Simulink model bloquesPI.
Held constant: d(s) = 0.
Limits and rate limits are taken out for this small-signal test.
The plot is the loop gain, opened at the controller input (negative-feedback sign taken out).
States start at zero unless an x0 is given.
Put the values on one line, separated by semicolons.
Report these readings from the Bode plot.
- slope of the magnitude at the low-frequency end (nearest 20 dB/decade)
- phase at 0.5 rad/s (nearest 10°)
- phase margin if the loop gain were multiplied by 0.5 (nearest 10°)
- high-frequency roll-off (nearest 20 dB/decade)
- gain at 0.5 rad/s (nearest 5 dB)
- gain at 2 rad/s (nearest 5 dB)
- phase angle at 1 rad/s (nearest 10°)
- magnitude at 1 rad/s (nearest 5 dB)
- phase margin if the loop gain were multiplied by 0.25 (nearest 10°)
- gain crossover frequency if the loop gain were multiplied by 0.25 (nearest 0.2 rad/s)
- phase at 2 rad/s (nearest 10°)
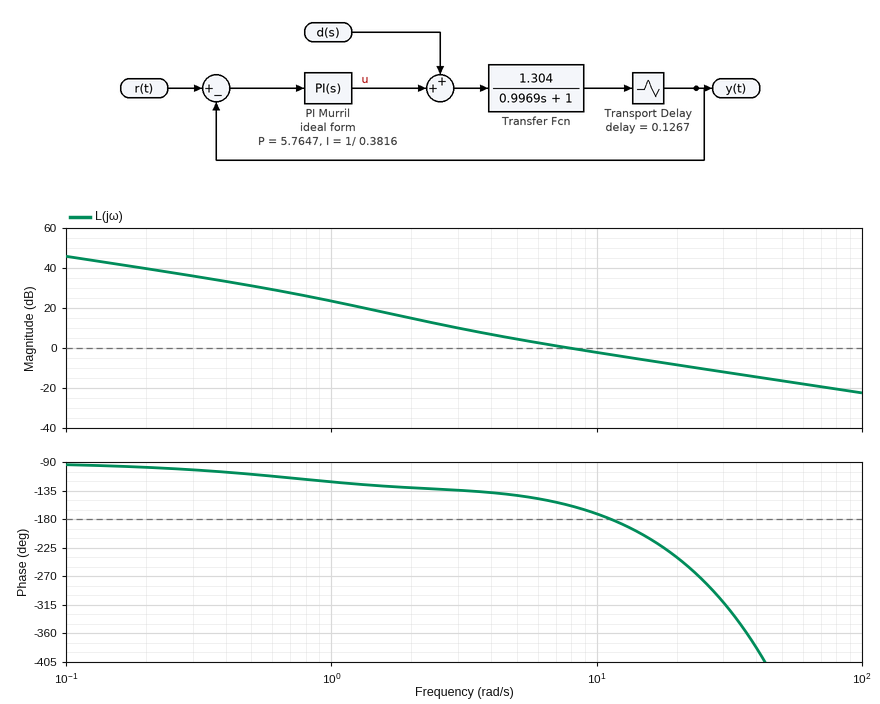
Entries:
-20 dB/decade; -110°; 40°; -20 dB/decade; 30 dB; 15 dB; -120°; 25 dB; 50°; 2.6 rad/s; -130°
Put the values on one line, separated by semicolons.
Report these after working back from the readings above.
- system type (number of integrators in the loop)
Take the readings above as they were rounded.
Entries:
1
